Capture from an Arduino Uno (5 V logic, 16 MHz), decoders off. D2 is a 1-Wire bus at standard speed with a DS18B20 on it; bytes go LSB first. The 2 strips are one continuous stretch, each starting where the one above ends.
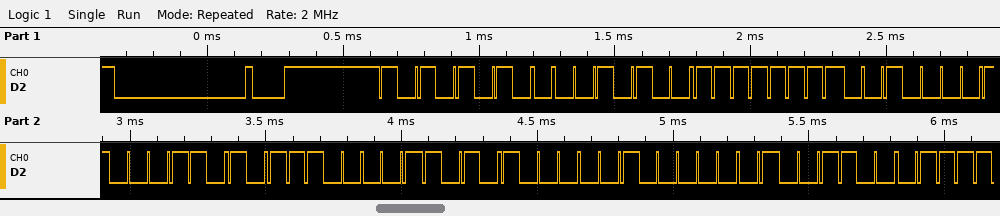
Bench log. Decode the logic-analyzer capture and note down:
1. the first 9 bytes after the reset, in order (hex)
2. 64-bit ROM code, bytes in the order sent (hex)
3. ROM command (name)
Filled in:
55 28 FF 84 58 87 15 04 32
28 FF 84 58 87 15 04 32
Match ROM
